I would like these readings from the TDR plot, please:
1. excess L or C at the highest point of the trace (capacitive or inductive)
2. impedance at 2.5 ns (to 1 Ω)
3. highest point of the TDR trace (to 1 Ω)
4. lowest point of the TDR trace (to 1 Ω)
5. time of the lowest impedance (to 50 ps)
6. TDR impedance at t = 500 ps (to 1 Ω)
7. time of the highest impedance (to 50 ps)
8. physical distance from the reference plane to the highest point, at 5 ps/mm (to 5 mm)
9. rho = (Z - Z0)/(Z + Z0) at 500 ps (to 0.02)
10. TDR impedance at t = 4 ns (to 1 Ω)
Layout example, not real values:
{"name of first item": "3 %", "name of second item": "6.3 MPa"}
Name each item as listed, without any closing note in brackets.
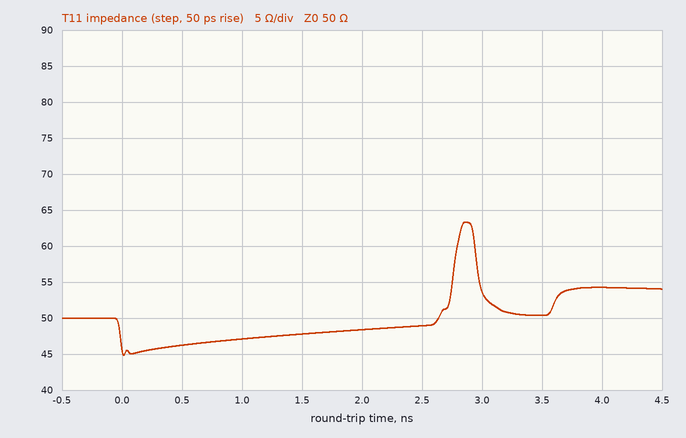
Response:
{"excess L or C at the highest point of the trace": "inductive", "impedance at 2.5 ns": "49 Ω", "highest point of the TDR trace": "63 Ω", "lowest point of the TDR trace": "45 Ω", "time of the lowest impedance": "0 ps", "TDR impedance at t = 500 ps": "46 Ω", "time of the highest impedance": "2.85 ns", "physical distance from the reference plane to the highest point, at 5 ps/mm": "285 mm", "rho = (Z - Z0)/(Z + Z0) at 500 ps": "-0.04", "TDR impedance at t = 4 ns": "54 Ω"}
